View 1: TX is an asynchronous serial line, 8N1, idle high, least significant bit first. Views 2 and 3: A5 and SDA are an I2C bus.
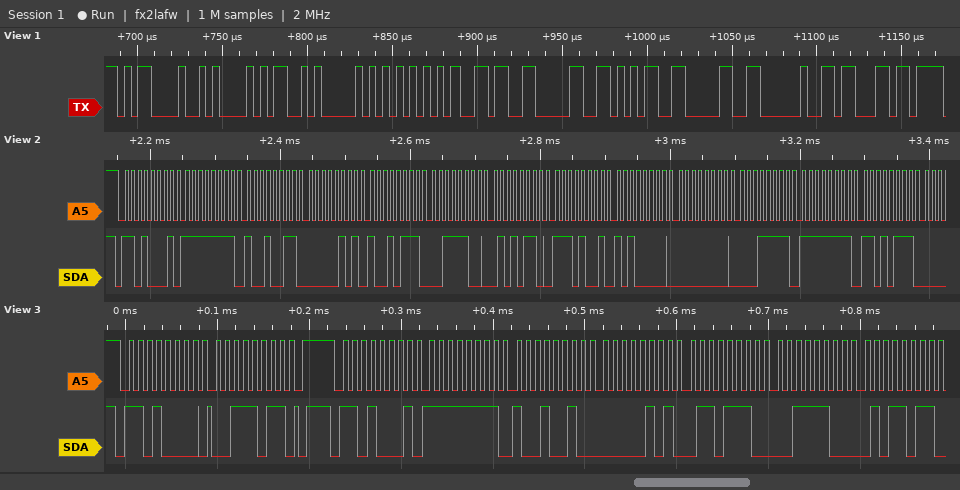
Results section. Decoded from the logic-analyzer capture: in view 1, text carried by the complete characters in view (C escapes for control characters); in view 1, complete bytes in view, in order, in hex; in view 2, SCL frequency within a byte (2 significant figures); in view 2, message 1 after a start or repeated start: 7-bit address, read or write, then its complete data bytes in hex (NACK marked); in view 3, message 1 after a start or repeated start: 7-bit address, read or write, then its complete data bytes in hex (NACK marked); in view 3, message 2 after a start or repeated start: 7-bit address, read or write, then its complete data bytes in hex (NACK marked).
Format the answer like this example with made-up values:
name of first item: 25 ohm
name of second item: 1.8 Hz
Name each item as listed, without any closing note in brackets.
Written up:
in view 1, text carried by the complete characters in view: "\r\nMPU6050 c"
in view 1, complete bytes in view, in order, in hex: 0D 0A 4D 50 55 36 30 35 30 20 63
in view 2, SCL frequency within a byte: 100 kHz
in view 2, message 1 after a start or repeated start: 7-bit address, read or write, then its complete data bytes in hex: 0x68 read: FF 93 05 97 3C 56 E9 A0 00 1F FF D7
in view 3, message 1 after a start or repeated start: 7-bit address, read or write, then its complete data bytes in hex: 0x68 write: 3B
in view 3, message 2 after a start or repeated start: 7-bit address, read or write, then its complete data bytes in hex: 0x68 read: FF 92 05 6E 3C 5B
